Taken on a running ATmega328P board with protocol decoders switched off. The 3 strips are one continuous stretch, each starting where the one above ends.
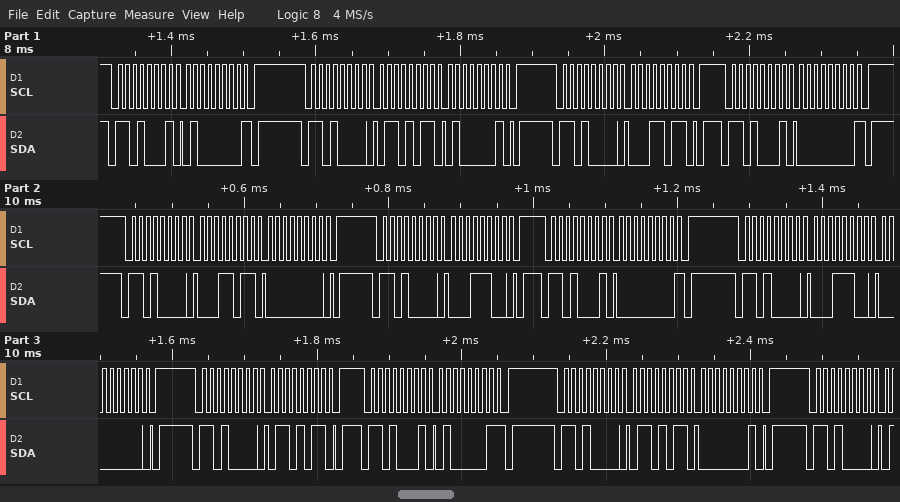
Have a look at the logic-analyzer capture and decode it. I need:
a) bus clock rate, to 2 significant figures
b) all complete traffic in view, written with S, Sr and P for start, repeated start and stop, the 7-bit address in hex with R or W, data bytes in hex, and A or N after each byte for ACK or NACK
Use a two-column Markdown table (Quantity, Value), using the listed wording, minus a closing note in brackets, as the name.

| Quantity | Value |
|---|---|
| bus clock rate, to 2 significant figures | 100 kHz |
| all complete traffic in view, written with S, Sr and P for start, repeated start and stop, the 7-bit address in hex with R or W, data bytes in hex, and A or N after each byte for ACK or NACK | S 68R A 40 N P S 68W A 6B A 41 A P S 68W A 1B A P S 68R A 00 N P S 68W A 1B A 00 A P S 68W A 1C A P S 68R A 00 N P S 68W A 1C A 00 A P S 68W A 6B A P S 68R A 41 N P S 68W A 6B A 01 A P S 68W A |
